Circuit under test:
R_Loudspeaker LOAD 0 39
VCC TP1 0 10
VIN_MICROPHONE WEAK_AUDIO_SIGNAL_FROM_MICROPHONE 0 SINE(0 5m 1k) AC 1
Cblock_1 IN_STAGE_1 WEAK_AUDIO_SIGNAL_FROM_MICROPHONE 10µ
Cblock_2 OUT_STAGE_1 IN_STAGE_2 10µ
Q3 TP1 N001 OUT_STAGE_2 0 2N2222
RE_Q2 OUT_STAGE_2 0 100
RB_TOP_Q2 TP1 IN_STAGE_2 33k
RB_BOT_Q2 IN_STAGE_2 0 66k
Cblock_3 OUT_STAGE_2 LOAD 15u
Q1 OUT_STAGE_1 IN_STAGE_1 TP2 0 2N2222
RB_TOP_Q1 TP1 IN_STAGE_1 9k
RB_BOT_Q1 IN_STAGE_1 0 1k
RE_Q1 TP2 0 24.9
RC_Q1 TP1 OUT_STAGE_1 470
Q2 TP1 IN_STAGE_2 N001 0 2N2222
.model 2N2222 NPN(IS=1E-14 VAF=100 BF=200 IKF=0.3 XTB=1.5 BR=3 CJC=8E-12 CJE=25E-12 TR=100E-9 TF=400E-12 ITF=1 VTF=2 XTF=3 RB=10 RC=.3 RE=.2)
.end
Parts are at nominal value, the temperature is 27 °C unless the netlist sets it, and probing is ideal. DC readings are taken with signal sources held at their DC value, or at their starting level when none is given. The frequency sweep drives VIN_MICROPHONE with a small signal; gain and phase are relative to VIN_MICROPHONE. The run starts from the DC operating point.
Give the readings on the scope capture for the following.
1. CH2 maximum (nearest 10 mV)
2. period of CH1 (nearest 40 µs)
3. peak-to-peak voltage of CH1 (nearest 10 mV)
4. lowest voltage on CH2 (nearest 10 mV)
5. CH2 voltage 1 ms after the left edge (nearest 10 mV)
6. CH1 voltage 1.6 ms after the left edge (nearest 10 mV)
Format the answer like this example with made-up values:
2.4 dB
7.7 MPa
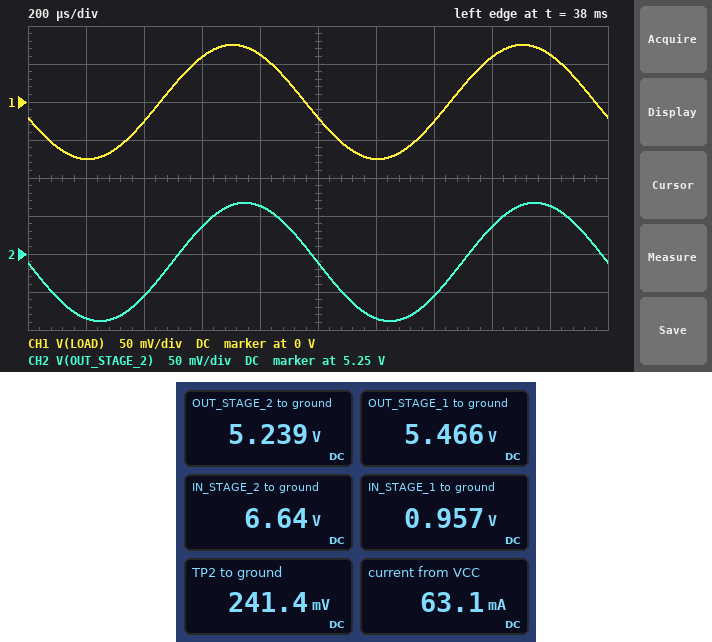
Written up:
5.32 V
1.00 ms
150 mV
5.16 V
5.24 V
60 mV
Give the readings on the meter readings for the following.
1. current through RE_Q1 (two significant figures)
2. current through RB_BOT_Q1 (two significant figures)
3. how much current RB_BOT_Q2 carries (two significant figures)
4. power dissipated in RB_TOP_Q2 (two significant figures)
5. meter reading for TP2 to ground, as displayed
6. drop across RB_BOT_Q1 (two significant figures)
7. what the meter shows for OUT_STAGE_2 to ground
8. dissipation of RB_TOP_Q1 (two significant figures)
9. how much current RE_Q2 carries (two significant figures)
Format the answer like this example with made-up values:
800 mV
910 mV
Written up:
9.7 mA
960 µA
100 µA
340 µW
241.4 mV
960 mV
5.239 V
9.1 mW
52 mA
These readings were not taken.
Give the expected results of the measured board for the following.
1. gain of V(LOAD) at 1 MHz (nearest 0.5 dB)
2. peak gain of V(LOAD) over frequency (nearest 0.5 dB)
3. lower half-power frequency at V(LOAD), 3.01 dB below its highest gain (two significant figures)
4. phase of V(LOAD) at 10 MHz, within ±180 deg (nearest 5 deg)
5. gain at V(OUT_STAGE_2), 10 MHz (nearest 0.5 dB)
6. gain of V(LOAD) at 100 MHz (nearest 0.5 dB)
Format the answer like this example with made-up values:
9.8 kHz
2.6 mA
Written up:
24.0 dB
24.0 dB
270 Hz
150 deg
24.0 dB
4.0 dB
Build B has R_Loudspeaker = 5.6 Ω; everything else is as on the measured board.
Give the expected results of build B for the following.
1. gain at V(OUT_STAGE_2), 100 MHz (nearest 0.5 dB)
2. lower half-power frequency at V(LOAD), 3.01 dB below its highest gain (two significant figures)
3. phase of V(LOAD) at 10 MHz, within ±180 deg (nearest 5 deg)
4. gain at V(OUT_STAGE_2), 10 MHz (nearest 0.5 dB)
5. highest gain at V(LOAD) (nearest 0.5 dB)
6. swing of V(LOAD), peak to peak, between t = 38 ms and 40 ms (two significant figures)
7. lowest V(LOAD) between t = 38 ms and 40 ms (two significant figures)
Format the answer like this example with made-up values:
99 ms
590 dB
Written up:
-6.5 dB
1.6 kHz
120 deg
21.5 dB
22.5 dB
71 mV
-35 mV
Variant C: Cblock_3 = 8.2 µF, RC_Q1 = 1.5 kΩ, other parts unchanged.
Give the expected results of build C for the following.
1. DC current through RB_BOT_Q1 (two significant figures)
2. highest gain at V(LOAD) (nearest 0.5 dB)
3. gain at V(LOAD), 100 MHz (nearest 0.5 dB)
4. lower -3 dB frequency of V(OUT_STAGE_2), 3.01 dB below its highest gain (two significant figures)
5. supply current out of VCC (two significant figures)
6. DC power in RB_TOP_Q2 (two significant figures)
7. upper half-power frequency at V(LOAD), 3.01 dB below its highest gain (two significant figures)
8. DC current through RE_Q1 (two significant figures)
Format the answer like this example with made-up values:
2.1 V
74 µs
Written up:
870 µA
11.0 dB
-6.0 dB
300 Hz
60 mA
340 µW
780 kHz
6.6 mA
